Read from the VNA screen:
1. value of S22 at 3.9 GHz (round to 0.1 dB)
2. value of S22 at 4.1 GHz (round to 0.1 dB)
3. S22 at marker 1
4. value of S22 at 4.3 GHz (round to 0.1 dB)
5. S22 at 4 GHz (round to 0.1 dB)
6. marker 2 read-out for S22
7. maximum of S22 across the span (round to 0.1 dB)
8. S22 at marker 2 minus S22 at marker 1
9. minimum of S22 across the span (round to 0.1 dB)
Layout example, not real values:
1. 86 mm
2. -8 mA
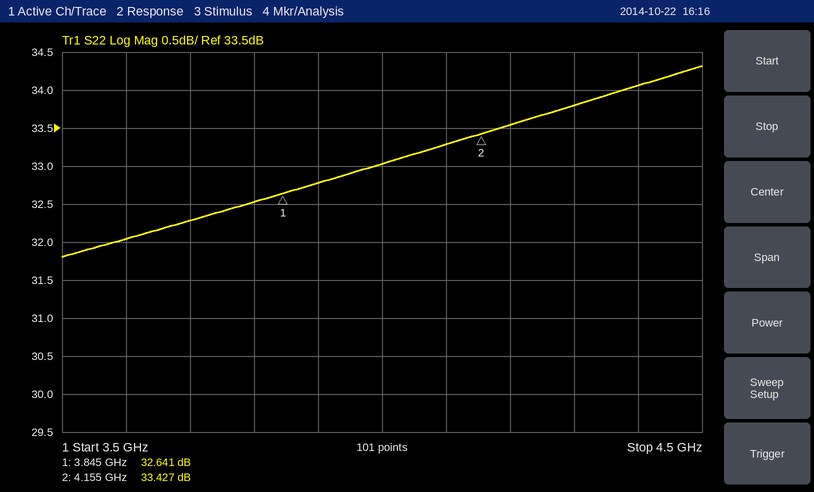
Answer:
1. 32.8 dB
2. 33.3 dB
3. 32.641 dB
4. 33.8 dB
5. 33.0 dB
6. 33.427 dB
7. 34.3 dB
8. 0.786 dB
9. 31.8 dB
